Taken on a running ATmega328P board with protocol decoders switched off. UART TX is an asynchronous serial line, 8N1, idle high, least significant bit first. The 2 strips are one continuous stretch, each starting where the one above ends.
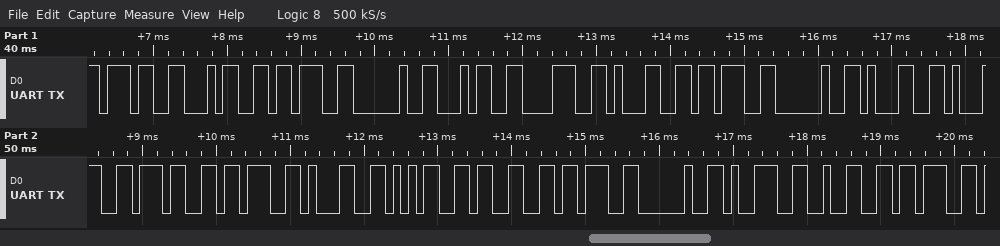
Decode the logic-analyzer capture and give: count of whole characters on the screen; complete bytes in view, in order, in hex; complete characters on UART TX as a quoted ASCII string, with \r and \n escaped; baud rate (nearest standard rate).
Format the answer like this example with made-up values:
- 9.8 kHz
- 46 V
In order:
- 21
- 37 34 3B 20 34 38 31 3B 20 31 31 37 3B 31 35 33 3B 20 39 32 3B
- "74; 481; 117;153; 92;"
- 9600 baud
